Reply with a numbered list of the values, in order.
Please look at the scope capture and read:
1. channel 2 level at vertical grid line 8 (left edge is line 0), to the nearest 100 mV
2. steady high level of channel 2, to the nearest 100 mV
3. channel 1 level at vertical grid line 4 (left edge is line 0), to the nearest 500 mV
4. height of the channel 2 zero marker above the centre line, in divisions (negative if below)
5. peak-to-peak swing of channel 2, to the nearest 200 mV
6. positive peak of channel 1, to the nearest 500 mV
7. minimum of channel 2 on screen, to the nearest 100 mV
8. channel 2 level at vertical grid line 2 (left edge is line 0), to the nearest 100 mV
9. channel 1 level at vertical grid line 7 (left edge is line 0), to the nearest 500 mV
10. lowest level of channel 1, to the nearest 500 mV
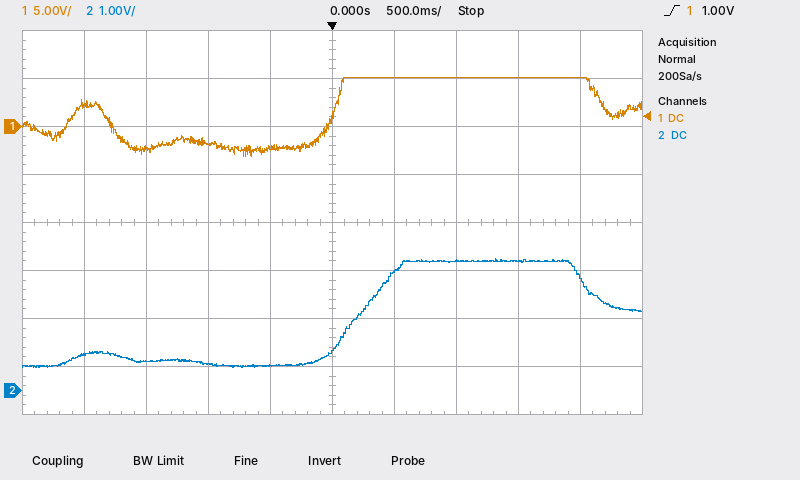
1. 2.7 V
2. 2.7 V
3. -2.5 V
4. -3.5 div
5. 2.2 V
6. 5.0 V
7. 500 mV
8. 600 mV
9. 5.0 V
10. -3.0 V
